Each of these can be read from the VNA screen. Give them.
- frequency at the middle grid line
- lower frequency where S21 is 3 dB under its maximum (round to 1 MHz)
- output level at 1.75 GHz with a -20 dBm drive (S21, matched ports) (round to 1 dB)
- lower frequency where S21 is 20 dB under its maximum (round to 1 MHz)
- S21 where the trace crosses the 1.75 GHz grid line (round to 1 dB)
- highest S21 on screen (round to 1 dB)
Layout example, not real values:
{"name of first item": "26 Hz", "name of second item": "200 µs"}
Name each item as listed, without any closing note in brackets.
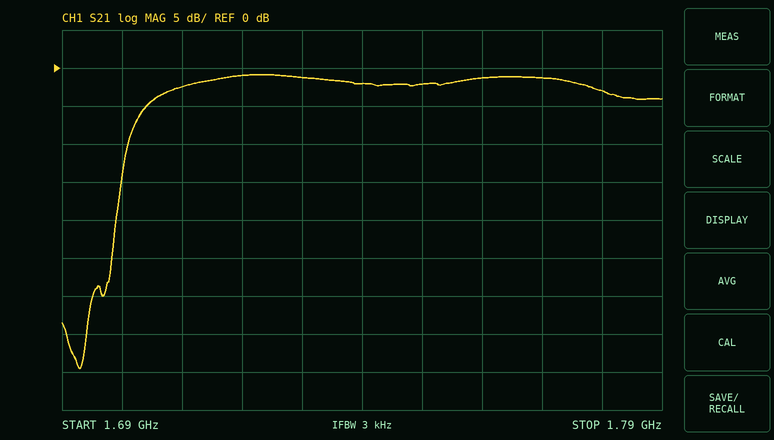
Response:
{"frequency at the middle grid line": "1.74 GHz", "lower frequency where S21 is 3 dB under its maximum": "1.706 GHz", "output level at 1.75 GHz with a -20 dBm drive (S21, matched ports)": "-22 dBm", "lower frequency where S21 is 20 dB under its maximum": "1.699 GHz", "S21 where the trace crosses the 1.75 GHz grid line": "-2 dB", "highest S21 on screen": "-1 dB"}
